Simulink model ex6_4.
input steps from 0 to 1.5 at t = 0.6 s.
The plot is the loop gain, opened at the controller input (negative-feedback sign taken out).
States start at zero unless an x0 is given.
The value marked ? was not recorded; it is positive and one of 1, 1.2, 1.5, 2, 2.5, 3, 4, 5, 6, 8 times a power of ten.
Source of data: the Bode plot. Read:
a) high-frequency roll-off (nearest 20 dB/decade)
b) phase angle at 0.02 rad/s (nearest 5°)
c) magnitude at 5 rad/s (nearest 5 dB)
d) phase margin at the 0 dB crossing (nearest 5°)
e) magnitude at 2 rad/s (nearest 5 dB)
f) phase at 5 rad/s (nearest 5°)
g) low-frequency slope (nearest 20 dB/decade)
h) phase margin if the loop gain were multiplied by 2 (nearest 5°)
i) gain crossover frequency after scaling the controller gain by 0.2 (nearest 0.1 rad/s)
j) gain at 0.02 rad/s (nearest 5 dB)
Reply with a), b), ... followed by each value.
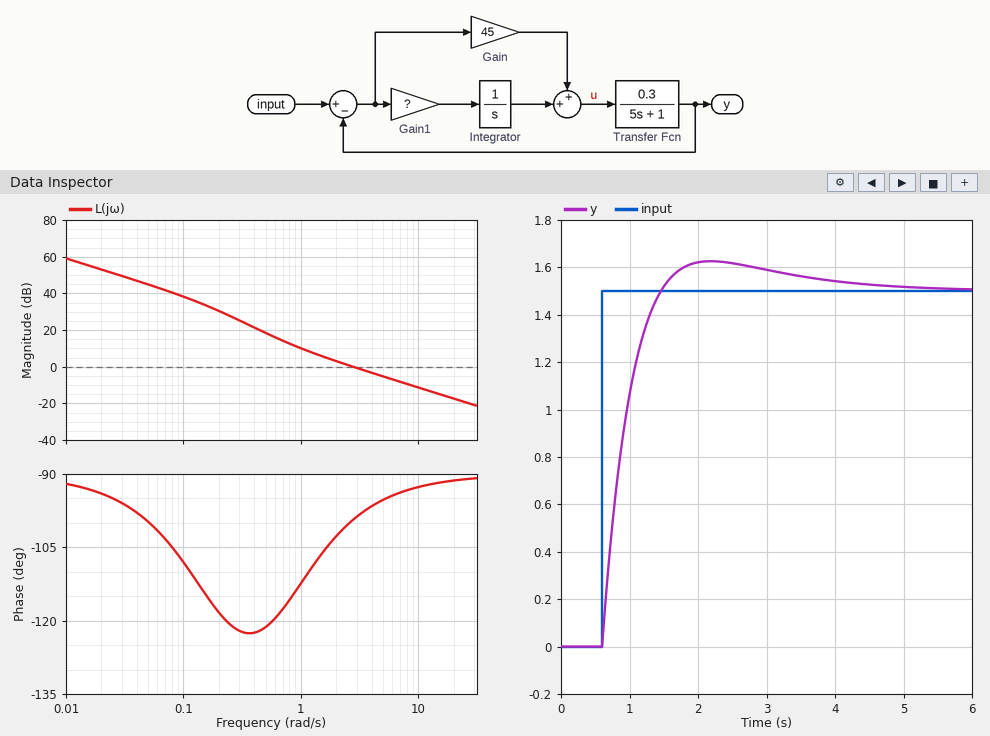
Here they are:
a) -20 dB/decade
b) -95°
c) -5 dB
d) 80°
e) 5 dB
f) -95°
g) -20 dB/decade
h) 85°
i) 0.7 rad/s
j) 55 dB
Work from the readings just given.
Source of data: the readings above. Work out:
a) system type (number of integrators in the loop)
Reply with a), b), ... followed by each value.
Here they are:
a) 1
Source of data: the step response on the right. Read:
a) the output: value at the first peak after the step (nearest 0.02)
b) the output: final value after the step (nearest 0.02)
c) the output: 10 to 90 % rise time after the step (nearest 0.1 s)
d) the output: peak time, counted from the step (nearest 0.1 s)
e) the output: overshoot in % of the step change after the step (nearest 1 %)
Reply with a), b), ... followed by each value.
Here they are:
a) 1.62
b) 1.50
c) 0.6 s
d) 1.6 s
e) 8 %
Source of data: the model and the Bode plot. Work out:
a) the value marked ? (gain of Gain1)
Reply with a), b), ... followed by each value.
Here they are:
a) 30
